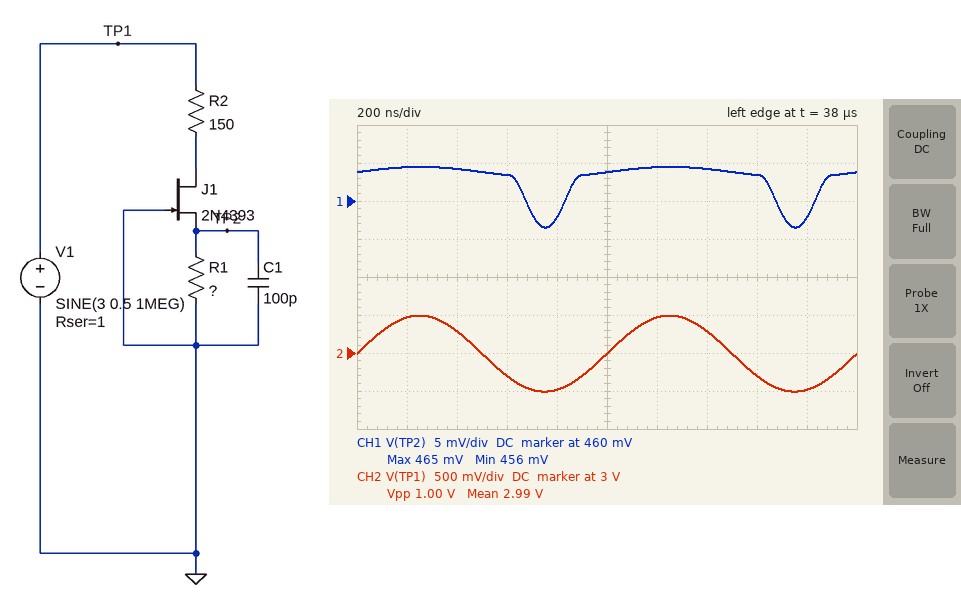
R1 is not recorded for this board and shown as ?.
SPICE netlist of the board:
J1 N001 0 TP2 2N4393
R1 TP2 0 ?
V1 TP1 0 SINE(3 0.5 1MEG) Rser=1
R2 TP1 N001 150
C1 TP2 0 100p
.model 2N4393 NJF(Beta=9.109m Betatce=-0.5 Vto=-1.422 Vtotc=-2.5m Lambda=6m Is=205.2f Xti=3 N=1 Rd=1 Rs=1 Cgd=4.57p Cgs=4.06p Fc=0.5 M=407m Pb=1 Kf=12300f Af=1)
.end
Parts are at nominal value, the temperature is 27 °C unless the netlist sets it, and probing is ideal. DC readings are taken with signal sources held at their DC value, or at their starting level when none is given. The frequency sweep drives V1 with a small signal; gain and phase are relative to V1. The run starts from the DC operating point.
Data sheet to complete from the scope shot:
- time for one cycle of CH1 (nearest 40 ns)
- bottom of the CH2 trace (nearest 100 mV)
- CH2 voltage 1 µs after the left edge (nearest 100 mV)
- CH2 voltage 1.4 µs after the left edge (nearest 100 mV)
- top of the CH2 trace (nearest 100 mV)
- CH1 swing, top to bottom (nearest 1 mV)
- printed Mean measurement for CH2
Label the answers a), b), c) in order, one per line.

a) 1.00 µs
b) 2.5 V
c) 3.0 V
d) 3.3 V
e) 3.5 V
f) 8 mV
g) 2.99 V
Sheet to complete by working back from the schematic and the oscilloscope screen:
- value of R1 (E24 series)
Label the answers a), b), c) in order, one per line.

a) 56 Ω
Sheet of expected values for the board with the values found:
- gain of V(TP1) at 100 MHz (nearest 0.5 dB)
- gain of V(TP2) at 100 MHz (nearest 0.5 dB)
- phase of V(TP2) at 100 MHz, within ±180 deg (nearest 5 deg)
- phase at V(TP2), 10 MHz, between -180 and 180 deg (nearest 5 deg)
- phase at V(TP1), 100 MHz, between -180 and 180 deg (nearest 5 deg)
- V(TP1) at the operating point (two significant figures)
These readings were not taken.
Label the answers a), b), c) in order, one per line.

a) 0 dB
b) -64.0 dB
c) -75 deg
d) -10 deg
e) 0 deg
f) 3.0 V
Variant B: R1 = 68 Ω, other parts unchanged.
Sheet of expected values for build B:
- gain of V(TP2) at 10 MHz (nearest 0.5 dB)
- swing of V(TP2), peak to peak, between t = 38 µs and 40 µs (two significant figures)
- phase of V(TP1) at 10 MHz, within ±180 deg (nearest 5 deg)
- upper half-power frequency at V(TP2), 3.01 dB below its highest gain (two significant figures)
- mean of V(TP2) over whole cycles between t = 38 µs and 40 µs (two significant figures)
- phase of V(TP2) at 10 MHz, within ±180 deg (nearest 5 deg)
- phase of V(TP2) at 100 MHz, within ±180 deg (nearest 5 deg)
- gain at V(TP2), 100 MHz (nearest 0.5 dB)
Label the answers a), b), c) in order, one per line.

a) -57.0 dB
b) 2.4 mV
c) 0 deg
d) 47 MHz
e) 510 mV
f) -15 deg
g) -80 deg
h) -64.5 dB
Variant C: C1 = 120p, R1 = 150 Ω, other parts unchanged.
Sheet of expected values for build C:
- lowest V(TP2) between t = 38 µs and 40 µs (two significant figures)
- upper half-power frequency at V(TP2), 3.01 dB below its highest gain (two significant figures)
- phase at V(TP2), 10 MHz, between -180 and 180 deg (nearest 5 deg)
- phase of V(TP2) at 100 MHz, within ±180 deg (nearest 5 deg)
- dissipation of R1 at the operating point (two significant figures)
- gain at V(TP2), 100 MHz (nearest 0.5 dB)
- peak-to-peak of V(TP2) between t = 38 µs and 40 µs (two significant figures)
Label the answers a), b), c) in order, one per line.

a) 700 mV
b) 25 MHz
c) -25 deg
d) -90 deg
e) 3.3 mW
f) -69.5 dB
g) 1.4 mV
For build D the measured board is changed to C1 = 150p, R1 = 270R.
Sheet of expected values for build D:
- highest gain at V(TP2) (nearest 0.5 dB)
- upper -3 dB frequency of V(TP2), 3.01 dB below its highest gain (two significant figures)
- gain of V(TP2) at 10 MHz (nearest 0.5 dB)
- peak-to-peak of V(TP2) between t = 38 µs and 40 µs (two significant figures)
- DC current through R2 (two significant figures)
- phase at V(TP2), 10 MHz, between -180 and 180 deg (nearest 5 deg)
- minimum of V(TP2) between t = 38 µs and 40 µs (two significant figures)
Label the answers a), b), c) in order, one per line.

a) -58.0 dB
b) 15 MHz
c) -59.5 dB
d) 1.3 mV
e) 3.1 mA
f) -35 deg
g) 840 mV
